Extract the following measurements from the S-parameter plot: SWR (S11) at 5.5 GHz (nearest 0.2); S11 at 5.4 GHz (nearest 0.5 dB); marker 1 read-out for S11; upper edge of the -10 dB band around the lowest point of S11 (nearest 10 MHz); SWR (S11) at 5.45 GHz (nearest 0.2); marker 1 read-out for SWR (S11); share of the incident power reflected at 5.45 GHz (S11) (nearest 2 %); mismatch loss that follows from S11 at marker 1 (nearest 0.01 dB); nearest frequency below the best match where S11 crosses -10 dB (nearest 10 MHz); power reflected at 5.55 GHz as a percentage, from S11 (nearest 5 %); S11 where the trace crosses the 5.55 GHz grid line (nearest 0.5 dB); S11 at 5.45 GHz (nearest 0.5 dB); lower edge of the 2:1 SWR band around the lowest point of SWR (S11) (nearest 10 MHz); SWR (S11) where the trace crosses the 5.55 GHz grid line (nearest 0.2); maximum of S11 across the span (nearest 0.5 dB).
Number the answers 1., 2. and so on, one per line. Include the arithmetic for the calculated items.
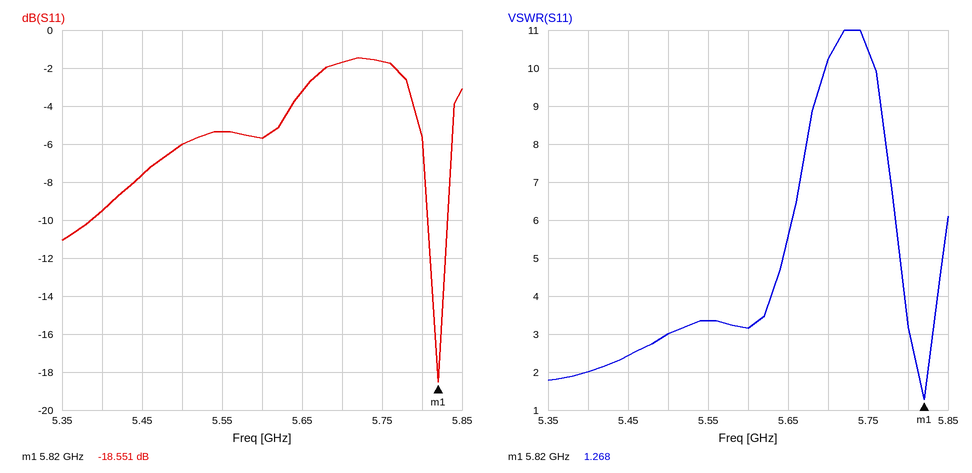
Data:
1. 3.0
2. -9.5 dB
3. -18.551 dB
4. 5.83 GHz
5. 2.4
6. 1.268
7. 10^(-7.5/10) ≈ 18 %
8. −10 log10(1 − 10^(-18.551/10)) ≈ 0.06 dB
9. 5.81 GHz
10. 10^(-5.5/10) ≈ 28.2 %, so 30 % to the nearest 5 %
11. -5.5 dB
12. -7.5 dB
13. 5.81 GHz
14. 3.4
15. -1.5 dB
